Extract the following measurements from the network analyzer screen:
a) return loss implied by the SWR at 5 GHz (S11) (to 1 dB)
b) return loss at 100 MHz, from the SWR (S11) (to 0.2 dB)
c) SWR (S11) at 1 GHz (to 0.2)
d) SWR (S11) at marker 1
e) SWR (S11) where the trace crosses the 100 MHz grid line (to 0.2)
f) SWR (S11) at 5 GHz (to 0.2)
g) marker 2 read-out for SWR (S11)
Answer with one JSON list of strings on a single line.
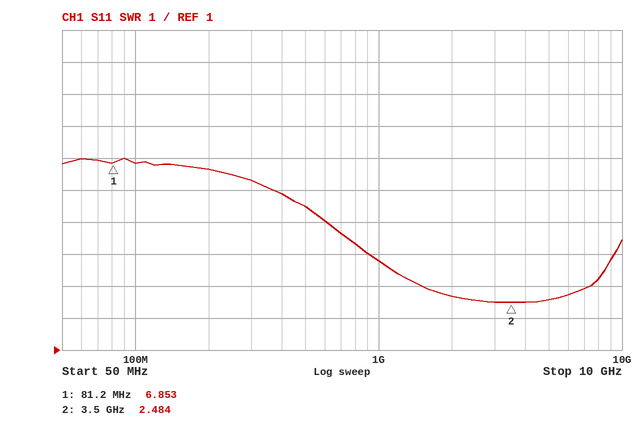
["7 dB", "2.6 dB", "3.8", "6.853", "6.8", "2.6", "2.484"]
